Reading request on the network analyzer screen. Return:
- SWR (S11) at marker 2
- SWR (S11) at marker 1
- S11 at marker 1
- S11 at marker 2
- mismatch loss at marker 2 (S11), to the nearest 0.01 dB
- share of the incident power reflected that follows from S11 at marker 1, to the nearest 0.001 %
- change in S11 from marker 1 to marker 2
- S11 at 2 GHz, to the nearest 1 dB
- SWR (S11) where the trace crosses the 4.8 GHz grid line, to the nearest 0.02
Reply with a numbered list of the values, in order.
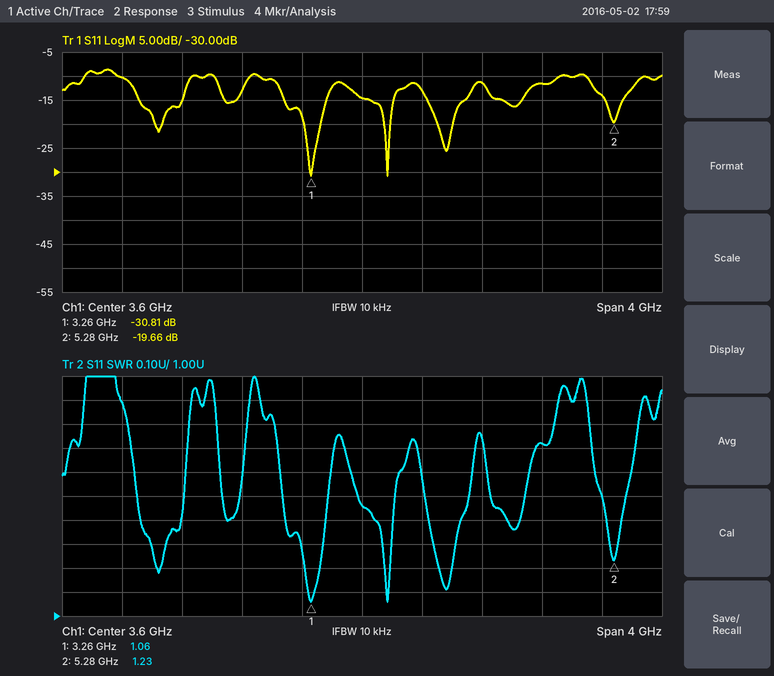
1. 1.23
2. 1.06
3. -30.81 dB
4. -19.66 dB
5. 0.05 dB
6. 0.083 %
7. 11.15 dB
8. -10 dB
9. 1.72
